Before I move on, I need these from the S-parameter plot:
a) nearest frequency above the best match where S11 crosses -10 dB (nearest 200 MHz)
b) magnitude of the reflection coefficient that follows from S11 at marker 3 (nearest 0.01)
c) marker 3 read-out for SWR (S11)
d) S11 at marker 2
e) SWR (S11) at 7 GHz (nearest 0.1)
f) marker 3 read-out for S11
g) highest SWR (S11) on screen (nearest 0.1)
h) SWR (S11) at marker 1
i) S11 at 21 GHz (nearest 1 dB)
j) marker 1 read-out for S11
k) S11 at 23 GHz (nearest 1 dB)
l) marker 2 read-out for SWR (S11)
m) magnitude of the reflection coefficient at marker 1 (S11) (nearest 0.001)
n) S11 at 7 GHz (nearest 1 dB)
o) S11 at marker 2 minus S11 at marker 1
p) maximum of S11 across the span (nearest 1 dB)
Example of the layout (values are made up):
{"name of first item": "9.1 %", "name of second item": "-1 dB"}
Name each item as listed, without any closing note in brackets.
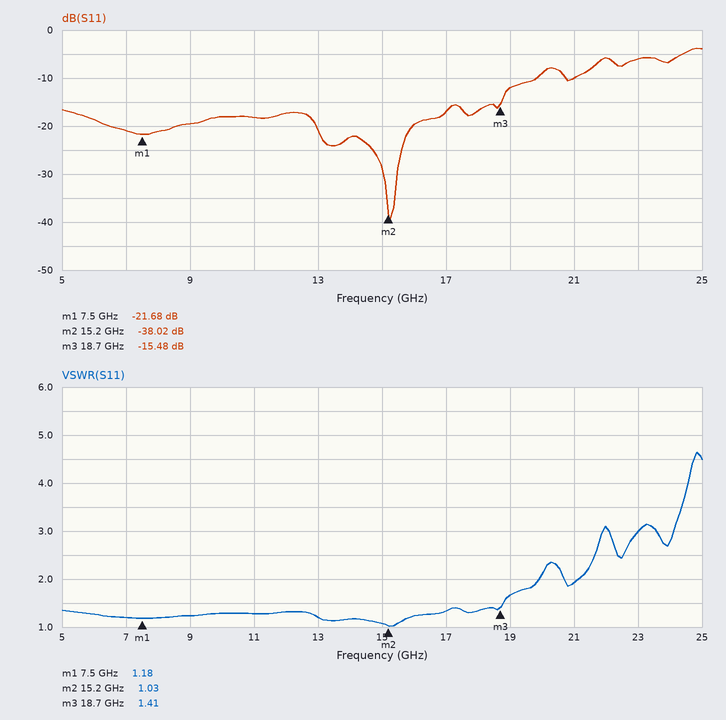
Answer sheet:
{"nearest frequency above the best match where S11 crosses -10 dB": "19.8 GHz", "magnitude of the reflection coefficient that follows from S11 at marker 3": "0.17", "marker 3 read-out for SWR": "1.41", "S11 at marker 2": "-38.02 dB", "SWR (S11) at 7 GHz": "1.2", "marker 3 read-out for S11": "-15.48 dB", "highest SWR (S11) on screen": "4.6", "SWR (S11) at marker 1": "1.18", "S11 at 21 GHz": "-10 dB", "marker 1 read-out for S11": "-21.68 dB", "S11 at 23 GHz": "-6 dB", "marker 2 read-out for SWR": "1.03", "magnitude of the reflection coefficient at marker 1 (S11)": "0.082", "S11 at 7 GHz": "-21 dB", "S11 at marker 2 minus S11 at marker 1": "-16.34 dB", "maximum of S11 across the span": "-4 dB"}
